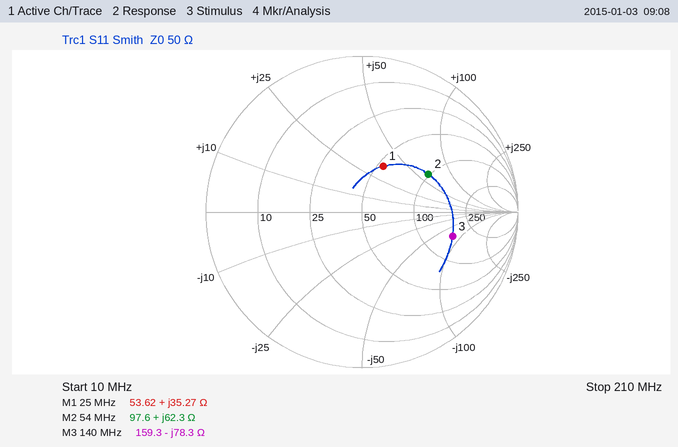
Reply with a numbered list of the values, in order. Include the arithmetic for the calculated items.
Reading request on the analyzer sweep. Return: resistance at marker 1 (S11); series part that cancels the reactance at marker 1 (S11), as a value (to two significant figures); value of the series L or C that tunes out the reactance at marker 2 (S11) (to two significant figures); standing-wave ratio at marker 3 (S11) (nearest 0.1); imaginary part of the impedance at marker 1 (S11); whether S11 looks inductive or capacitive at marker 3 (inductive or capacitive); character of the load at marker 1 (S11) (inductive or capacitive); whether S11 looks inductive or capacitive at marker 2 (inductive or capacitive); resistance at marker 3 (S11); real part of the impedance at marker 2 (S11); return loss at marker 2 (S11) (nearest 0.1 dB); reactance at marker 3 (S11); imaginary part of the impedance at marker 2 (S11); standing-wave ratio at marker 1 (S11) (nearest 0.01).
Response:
1. 53.62 Ω
2. C = 1/(2π × 25 MHz × 35.27 Ω) ≈ 180 pF
3. C = 1/(2π × 54 MHz × 62.3 Ω) ≈ 47 pF
4. 4.0
5. +35.27 Ω
6. capacitive
7. inductive
8. inductive
9. 159.3 Ω
10. 97.6 Ω
11. 6.2 dB
12. -78.3 Ω
13. +62.3 Ω
14. 1.96
